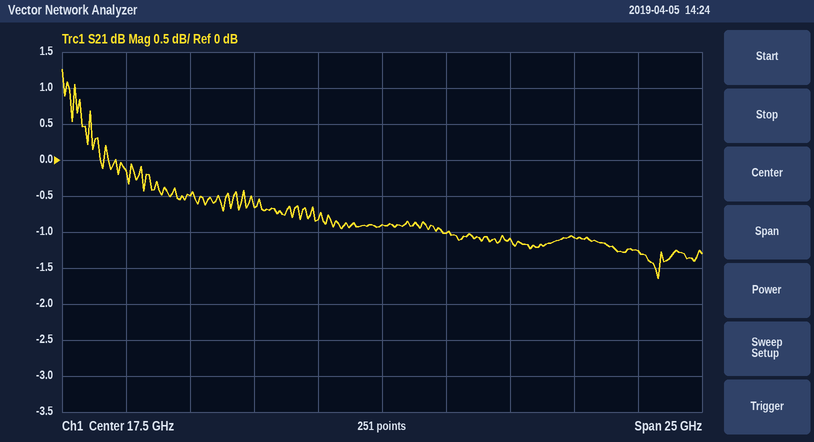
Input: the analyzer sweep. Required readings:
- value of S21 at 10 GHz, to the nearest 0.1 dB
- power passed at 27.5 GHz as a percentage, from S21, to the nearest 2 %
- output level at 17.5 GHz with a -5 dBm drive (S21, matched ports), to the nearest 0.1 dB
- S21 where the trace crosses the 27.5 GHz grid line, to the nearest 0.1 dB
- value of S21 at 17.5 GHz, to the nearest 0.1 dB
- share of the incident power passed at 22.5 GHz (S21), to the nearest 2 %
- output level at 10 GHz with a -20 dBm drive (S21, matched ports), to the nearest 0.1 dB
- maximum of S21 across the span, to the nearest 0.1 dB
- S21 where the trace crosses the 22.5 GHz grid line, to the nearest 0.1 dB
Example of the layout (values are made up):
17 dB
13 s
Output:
-0.5 dB
74 %
-5.9 dBm
-1.3 dB
-0.9 dB
78 %
-20.5 dBm
1.3 dB
-1.1 dB
